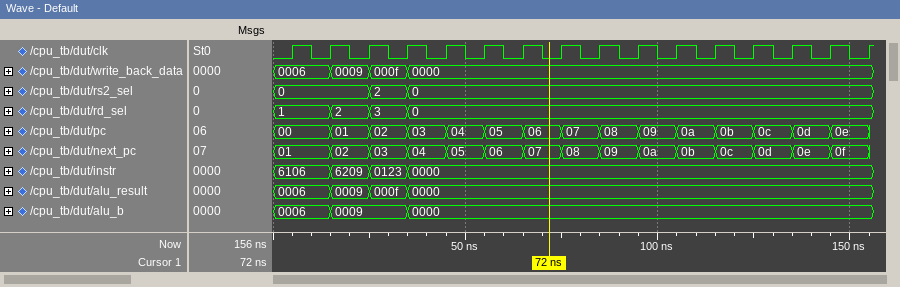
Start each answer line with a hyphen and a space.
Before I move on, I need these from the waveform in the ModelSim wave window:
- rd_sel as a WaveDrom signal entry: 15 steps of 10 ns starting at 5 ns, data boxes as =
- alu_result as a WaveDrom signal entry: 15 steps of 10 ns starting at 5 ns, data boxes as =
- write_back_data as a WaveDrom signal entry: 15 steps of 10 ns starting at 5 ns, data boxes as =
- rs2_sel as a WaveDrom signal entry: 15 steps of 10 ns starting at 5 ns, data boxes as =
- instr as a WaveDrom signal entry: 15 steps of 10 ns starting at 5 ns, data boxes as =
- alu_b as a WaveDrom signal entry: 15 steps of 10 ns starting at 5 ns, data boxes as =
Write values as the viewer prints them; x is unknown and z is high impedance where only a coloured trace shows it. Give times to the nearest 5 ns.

- {name: 'rd_sel', wave: '====...........', data: '1 2 3 0'}
- {name: 'alu_result', wave: '====...........', data: '0006 0009 000f 0000'}
- {name: 'write_back_data', wave: '====...........', data: '0006 0009 000f 0000'}
- {name: 'rs2_sel', wave: '=.==...........', data: '0 2 0'}
- {name: 'instr', wave: '====...........', data: '6106 6209 0123 0000'}
- {name: 'alu_b', wave: '==.=...........', data: '0006 0009 0000'}
